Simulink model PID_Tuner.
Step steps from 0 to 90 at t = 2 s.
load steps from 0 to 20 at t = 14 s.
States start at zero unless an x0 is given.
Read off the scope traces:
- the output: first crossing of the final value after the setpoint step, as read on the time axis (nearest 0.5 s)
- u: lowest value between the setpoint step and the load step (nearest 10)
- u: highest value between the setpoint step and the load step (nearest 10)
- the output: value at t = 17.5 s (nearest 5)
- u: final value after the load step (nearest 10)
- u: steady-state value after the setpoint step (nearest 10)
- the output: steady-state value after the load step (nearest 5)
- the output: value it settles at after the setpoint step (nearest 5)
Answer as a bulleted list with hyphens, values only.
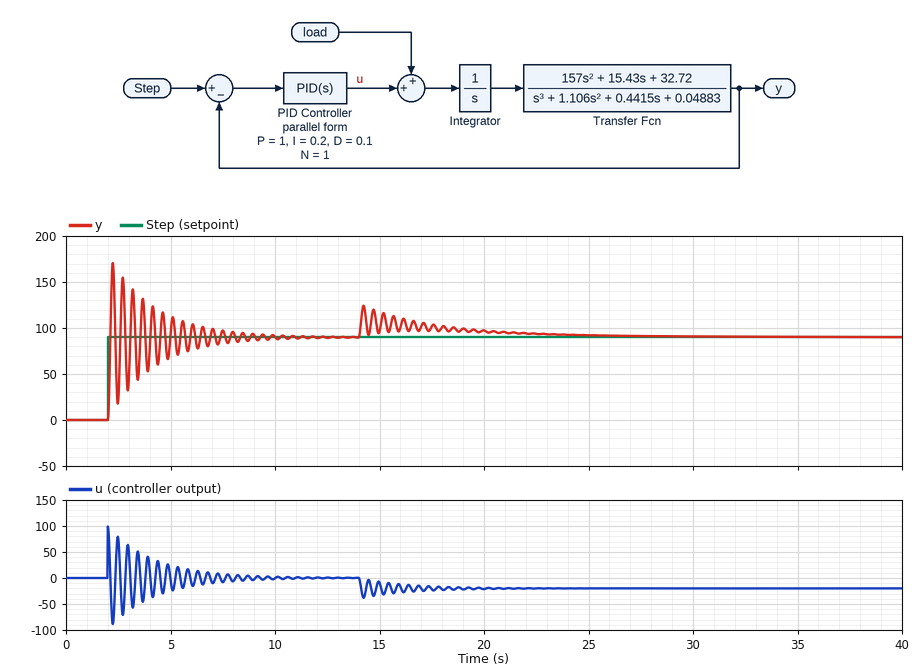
- 2.0 s
- -90
- 100
- 100
- -20
- 0
- 90
- 90
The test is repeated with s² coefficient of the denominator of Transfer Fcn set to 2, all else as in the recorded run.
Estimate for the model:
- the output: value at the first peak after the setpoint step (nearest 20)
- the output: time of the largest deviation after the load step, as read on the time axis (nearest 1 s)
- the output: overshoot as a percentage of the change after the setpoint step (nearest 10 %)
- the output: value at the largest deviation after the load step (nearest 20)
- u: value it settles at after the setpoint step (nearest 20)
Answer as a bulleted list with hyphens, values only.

- 160
- 14 s
- 80 %
- 120
- 0
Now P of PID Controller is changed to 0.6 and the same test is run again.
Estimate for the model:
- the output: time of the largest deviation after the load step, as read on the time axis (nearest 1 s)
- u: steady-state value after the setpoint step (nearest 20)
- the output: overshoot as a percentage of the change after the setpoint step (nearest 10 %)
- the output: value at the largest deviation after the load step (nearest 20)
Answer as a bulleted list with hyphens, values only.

- 14 s
- 0
- 90 %
- 140
